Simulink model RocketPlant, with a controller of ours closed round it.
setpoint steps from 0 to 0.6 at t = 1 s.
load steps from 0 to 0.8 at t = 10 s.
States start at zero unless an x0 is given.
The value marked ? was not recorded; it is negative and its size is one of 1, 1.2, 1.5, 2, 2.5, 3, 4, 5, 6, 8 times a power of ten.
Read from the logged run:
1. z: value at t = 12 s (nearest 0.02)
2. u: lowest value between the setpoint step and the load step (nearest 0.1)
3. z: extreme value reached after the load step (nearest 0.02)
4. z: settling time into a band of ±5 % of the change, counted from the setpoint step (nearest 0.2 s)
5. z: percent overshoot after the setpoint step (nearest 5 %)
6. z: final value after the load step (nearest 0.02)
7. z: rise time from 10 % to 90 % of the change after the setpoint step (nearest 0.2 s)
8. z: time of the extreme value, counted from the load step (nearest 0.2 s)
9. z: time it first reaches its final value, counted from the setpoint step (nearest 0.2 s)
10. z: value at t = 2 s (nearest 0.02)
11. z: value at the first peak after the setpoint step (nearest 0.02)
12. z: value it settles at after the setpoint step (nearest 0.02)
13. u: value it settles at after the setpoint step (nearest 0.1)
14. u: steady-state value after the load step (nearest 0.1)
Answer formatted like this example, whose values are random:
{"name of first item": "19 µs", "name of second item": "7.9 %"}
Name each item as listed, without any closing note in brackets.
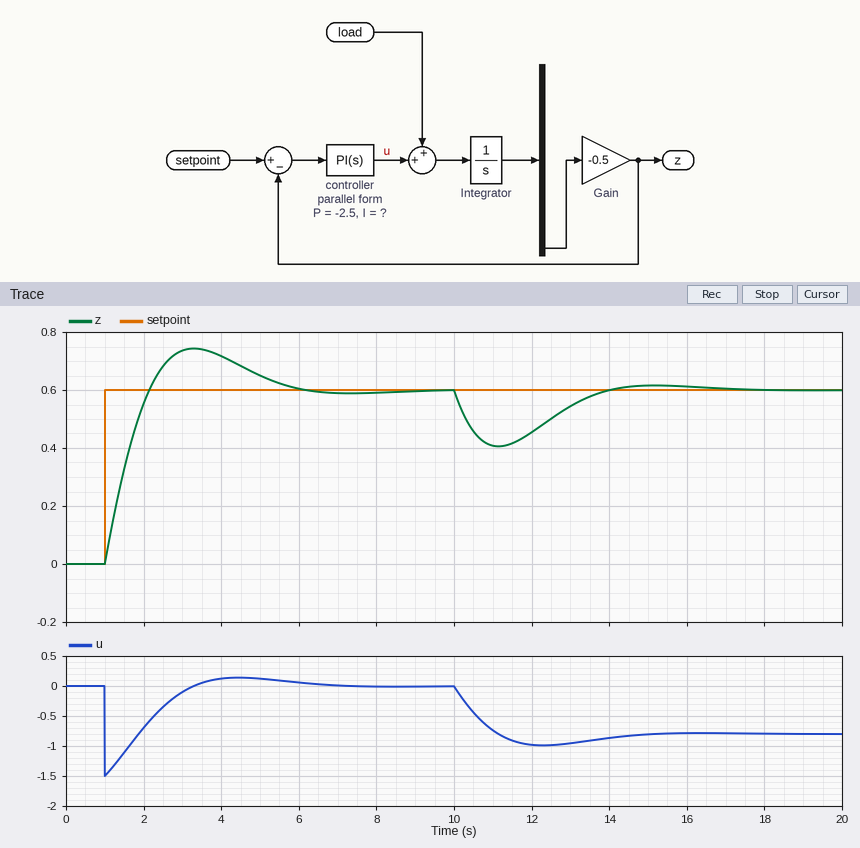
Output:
{"z: value at t = 12 s": "0.46", "u: lowest value between the setpoint step and the load step": "-1.5", "z: extreme value reached after the load step": "0.40", "z: settling time into a band of ±5 % of the change, counted from the setpoint step": "4.4 s", "z: percent overshoot after the setpoint step": "25 %", "z: final value after the load step": "0.60", "z: rise time from 10 % to 90 % of the change after the setpoint step": "0.8 s", "z: time of the extreme value, counted from the load step": "1.2 s", "z: time it first reaches its final value, counted from the setpoint step": "1.2 s", "z: value at t = 2 s": "0.56", "z: value at the first peak after the setpoint step": "0.74", "z: value it settles at after the setpoint step": "0.60", "u: value it settles at after the setpoint step": "0.0", "u: steady-state value after the load step": "-0.8"}
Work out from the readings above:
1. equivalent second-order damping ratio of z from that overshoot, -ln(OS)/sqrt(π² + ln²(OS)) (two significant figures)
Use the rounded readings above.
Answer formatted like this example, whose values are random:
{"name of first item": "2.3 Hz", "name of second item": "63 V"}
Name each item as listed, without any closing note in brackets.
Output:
{"equivalent second-order damping ratio of z from that overshoot, -ln(OS)/sqrt(π² + ln²(OS))": "0.40"}
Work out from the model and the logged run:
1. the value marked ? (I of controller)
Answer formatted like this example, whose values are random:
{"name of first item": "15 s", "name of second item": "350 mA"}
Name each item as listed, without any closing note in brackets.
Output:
{"the value marked ?": "-2"}
